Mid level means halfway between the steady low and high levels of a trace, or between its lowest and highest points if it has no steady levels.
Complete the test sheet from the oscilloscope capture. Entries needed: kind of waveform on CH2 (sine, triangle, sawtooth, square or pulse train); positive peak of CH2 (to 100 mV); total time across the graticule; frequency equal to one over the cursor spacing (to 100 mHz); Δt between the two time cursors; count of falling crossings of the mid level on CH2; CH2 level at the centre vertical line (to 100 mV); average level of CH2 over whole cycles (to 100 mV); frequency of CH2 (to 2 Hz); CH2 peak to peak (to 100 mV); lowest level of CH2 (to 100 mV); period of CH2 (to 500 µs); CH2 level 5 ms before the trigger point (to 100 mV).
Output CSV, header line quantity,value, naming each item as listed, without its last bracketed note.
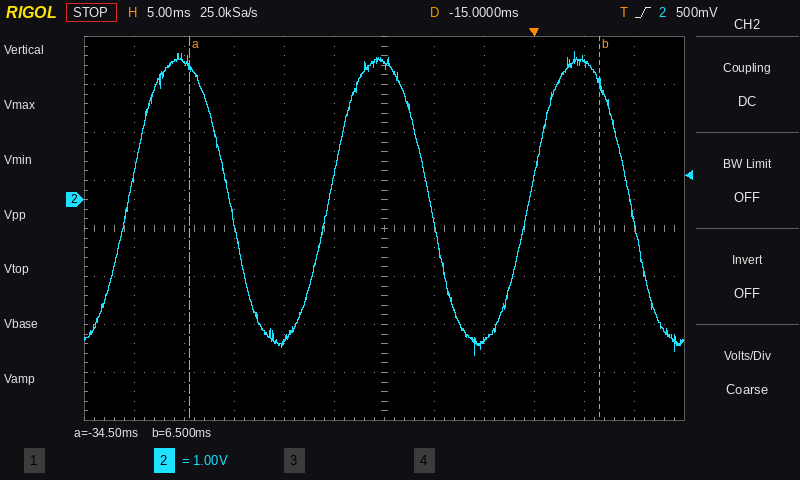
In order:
quantity,value
kind of waveform on CH2,sine
positive peak of CH2,3.1 V
total time across the graticule,60 ms
frequency equal to one over the cursor spacing,24.4 Hz
Δt between the two time cursors,41.0 ms
count of falling crossings of the mid level on CH2,3
CH2 level at the centre vertical line,2.8 V
average level of CH2 over whole cycles,0.0 V
frequency of CH2,50 Hz
CH2 peak to peak,6.3 V
lowest level of CH2,-3.2 V
period of CH2,20.0 ms
CH2 level 5 ms before the trigger point,-2.9 V
